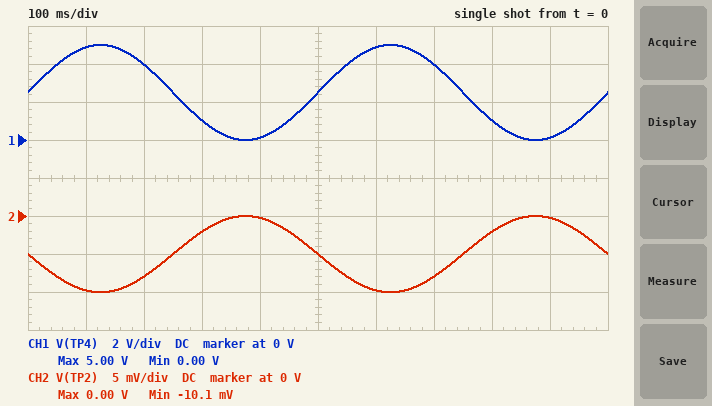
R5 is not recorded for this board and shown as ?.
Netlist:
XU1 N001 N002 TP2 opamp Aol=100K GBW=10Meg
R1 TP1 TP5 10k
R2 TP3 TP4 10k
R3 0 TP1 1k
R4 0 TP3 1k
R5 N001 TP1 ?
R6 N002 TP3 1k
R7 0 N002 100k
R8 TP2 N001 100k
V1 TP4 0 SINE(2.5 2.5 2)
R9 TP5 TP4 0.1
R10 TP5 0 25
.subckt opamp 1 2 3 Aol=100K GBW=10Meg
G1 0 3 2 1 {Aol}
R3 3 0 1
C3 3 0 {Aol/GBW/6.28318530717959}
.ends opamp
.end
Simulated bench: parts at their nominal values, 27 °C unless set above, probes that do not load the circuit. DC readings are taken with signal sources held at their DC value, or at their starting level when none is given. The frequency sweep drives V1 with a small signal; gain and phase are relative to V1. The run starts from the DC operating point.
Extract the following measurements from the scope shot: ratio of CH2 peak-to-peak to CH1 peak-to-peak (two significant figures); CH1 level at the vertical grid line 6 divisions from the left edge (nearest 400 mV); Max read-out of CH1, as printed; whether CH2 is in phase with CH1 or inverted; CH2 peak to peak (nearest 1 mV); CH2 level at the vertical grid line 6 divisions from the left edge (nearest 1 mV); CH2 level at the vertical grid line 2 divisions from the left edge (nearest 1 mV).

0.0020
4.8 V
5.00 V
inverted
10 mV
-10 mV
-8 mV
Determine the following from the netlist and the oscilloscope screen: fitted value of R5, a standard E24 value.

560 Ω
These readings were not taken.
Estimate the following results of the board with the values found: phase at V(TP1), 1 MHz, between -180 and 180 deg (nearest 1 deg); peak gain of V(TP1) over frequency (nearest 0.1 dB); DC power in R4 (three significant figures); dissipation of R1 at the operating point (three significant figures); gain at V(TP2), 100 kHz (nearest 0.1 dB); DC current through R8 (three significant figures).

0 deg
-20.9 dB
50.7 µW
513 µW
-55.6 dB
2.28 µA
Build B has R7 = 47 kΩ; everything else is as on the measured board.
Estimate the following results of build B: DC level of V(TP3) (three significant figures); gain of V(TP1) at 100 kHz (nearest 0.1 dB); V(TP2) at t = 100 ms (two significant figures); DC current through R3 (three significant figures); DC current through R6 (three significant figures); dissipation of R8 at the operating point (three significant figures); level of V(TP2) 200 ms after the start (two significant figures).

223 mV
-21.0 dB
-630 mV
221 µA
4.65 µA
2.94 µW
-510 mV
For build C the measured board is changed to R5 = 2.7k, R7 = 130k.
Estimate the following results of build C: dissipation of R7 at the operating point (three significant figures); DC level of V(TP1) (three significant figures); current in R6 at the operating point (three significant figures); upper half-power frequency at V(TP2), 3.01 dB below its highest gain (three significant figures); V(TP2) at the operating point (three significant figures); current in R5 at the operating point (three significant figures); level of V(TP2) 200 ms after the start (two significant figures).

386 nW
226 mV
1.72 µA
348 kHz
158 mV
660 nA
250 mV
